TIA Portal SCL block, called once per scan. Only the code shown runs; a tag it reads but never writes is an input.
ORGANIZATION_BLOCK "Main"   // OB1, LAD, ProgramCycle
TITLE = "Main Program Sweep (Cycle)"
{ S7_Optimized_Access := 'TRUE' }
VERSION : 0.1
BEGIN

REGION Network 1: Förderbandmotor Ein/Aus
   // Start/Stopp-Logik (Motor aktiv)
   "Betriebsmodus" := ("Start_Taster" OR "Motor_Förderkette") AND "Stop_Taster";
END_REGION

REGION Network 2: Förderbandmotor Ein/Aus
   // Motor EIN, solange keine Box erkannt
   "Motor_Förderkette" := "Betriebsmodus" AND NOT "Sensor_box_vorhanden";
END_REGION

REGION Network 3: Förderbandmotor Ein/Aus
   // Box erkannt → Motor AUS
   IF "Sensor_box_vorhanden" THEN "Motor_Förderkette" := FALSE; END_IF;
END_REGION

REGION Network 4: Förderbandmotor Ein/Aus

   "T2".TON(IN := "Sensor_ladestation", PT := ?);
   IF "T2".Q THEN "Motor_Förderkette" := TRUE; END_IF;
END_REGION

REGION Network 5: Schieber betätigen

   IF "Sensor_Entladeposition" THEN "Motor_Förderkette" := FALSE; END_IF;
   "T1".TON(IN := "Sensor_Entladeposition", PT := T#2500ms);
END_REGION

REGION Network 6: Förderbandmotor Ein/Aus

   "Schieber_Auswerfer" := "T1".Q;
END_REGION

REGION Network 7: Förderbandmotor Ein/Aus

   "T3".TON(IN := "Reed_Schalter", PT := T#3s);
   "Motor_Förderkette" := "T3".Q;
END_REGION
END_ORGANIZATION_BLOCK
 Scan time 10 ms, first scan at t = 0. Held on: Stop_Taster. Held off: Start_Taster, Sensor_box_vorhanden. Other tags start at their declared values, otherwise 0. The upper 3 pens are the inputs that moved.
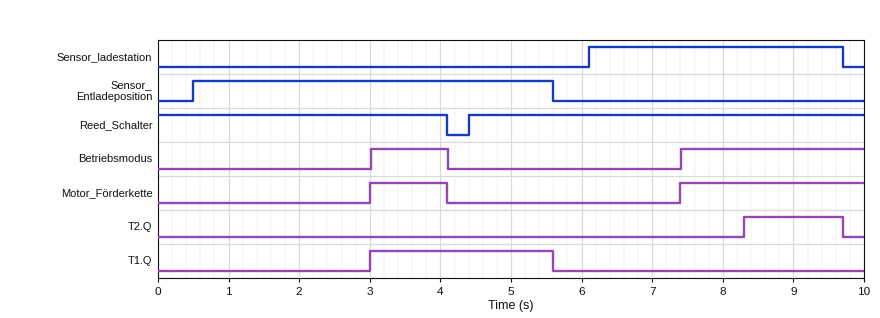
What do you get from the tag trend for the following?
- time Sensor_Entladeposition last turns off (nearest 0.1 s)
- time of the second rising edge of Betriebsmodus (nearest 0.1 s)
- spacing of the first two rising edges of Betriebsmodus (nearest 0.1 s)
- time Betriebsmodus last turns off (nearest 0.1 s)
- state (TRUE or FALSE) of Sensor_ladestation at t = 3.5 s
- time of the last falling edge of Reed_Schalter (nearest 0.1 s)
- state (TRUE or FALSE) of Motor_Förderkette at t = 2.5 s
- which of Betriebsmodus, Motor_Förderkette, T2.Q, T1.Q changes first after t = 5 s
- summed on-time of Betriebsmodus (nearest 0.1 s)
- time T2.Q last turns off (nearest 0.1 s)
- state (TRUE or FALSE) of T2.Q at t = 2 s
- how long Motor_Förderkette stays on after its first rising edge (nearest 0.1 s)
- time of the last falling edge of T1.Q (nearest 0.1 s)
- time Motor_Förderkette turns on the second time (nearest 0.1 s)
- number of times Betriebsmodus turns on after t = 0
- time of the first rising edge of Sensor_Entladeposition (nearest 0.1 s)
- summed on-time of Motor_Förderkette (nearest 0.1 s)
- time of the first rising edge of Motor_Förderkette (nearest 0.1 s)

5.6 s
7.4 s
4.4 s
4.1 s
FALSE
4.1 s
FALSE
T1.Q
3.7 s
9.7 s
FALSE
1.1 s
5.6 s
7.4 s
2
0.5 s
3.7 s
3.0 s
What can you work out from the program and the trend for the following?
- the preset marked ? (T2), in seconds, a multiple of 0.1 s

2.2 s
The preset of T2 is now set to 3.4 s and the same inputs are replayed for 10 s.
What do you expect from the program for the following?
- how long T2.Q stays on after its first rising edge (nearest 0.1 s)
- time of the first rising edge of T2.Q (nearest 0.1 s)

0.2 s
9.5 s
